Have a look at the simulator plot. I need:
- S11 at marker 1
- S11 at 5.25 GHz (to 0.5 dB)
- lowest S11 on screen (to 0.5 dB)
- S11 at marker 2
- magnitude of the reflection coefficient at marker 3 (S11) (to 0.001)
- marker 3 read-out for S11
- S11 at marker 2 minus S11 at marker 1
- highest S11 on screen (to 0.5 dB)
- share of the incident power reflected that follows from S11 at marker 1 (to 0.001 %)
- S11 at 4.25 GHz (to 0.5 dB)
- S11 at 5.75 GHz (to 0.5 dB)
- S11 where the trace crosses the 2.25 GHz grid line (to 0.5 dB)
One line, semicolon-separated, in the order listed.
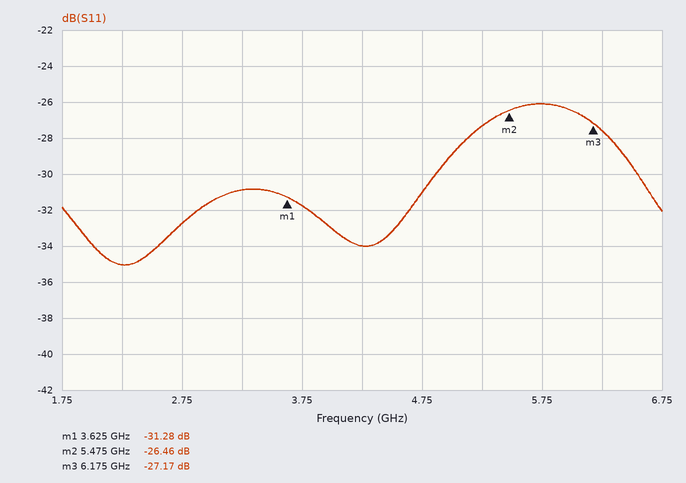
-31.28 dB; -27.5 dB; -35.0 dB; -26.46 dB; 0.044; -27.17 dB; 4.82 dB; -26.0 dB; 0.074 %; -34.0 dB; -26.0 dB; -35.0 dB
